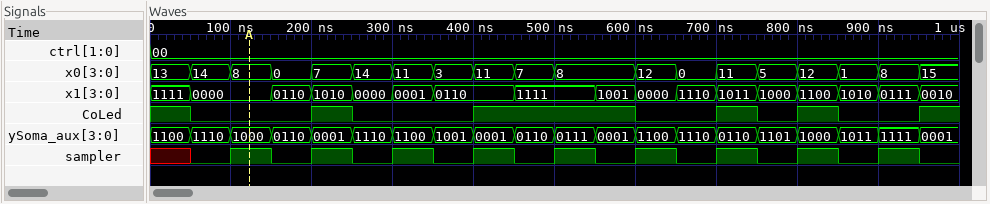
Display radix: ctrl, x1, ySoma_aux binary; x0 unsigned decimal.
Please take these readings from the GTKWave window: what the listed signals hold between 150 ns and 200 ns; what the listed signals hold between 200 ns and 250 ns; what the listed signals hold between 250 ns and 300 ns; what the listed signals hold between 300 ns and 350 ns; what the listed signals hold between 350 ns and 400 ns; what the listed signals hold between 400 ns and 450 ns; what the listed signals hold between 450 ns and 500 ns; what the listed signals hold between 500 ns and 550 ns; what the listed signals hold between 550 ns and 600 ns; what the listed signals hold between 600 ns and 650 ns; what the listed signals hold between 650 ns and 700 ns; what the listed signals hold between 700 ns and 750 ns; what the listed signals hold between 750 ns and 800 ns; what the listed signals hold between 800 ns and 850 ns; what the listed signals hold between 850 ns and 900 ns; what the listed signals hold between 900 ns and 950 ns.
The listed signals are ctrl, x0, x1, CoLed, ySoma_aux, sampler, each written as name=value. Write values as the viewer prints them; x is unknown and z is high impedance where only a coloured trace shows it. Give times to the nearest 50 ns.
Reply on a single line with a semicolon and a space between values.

ctrl=00, x0=0, x1=0110, CoLed=0, ySoma_aux=0110, sampler=0; ctrl=00, x0=7, x1=1010, CoLed=1, ySoma_aux=0001, sampler=1; ctrl=00, x0=14, x1=0000, CoLed=0, ySoma_aux=1110, sampler=0; ctrl=00, x0=11, x1=0001, CoLed=0, ySoma_aux=1100, sampler=1; ctrl=00, x0=3, x1=0110, CoLed=0, ySoma_aux=1001, sampler=0; ctrl=00, x0=11, x1=0110, CoLed=1, ySoma_aux=0001, sampler=1; ctrl=00, x0=7, x1=1111, CoLed=1, ySoma_aux=0110, sampler=0; ctrl=00, x0=8, x1=1111, CoLed=1, ySoma_aux=0111, sampler=1; ctrl=00, x0=8, x1=1001, CoLed=1, ySoma_aux=0001, sampler=0; ctrl=00, x0=12, x1=0000, CoLed=0, ySoma_aux=1100, sampler=1; ctrl=00, x0=0, x1=1110, CoLed=0, ySoma_aux=1110, sampler=0; ctrl=00, x0=11, x1=1011, CoLed=1, ySoma_aux=0110, sampler=1; ctrl=00, x0=5, x1=1000, CoLed=0, ySoma_aux=1101, sampler=0; ctrl=00, x0=12, x1=1100, CoLed=1, ySoma_aux=1000, sampler=1; ctrl=00, x0=1, x1=1010, CoLed=0, ySoma_aux=1011, sampler=0; ctrl=00, x0=8, x1=0111, CoLed=0, ySoma_aux=1111, sampler=1
